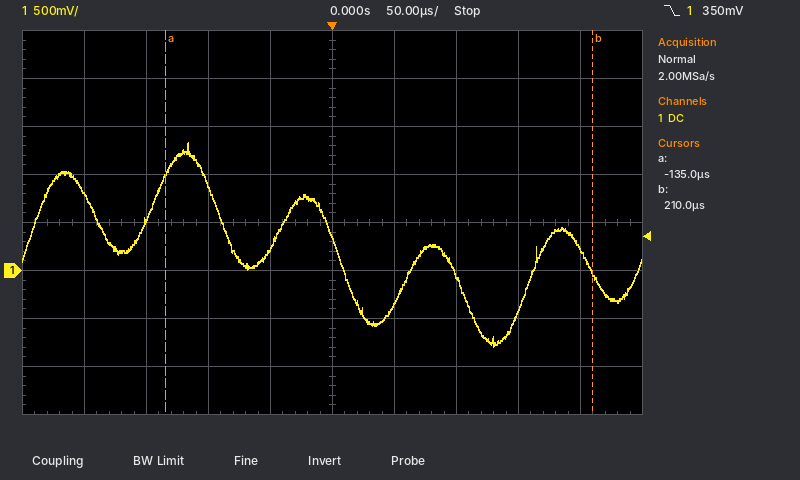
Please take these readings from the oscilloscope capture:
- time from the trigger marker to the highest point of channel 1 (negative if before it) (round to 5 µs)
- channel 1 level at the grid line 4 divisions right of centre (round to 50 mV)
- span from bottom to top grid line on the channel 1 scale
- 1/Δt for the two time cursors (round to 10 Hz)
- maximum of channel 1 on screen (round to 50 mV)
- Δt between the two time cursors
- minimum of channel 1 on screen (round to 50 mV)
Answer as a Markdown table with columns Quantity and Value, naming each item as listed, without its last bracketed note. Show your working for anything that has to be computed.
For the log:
| Quantity | Value |
|---|---|
| time from the trigger marker to the highest point of channel 1 (negative if before it) | -115 µs |
| channel 1 level at the grid line 4 divisions right of centre | 250 mV |
| span from bottom to top grid line on the channel 1 scale | 4 V |
| 1/Δt for the two time cursors | 1 / 345 µs ≈ 2.90 kHz |
| maximum of channel 1 on screen | 1.35 V |
| Δt between the two time cursors | 210 µs − (-135 µs) = 345 µs |
| minimum of channel 1 on screen | -800 mV |
